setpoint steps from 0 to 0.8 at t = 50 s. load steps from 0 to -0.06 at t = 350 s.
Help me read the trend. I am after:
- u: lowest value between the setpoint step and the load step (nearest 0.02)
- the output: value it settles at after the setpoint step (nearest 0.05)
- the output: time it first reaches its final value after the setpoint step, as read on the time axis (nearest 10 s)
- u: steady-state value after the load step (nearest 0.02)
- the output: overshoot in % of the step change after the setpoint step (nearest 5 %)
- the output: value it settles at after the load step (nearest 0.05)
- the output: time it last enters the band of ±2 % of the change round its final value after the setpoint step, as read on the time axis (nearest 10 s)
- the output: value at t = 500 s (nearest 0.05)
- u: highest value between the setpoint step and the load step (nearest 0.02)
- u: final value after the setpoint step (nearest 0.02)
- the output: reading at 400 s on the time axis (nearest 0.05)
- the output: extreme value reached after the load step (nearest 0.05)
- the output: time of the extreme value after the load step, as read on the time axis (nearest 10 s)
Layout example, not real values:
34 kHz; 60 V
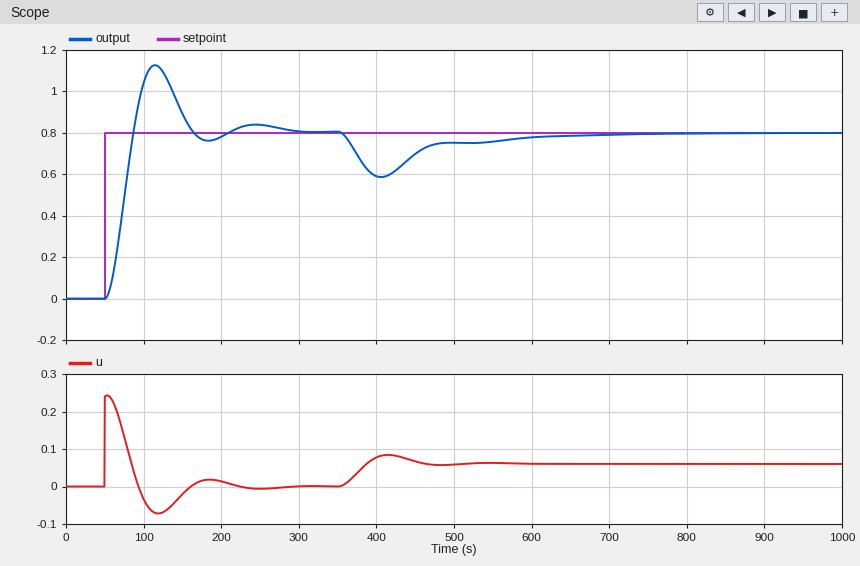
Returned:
-0.08; 0.80; 90 s; 0.06; 40 %; 0.80; 280 s; 0.75; 0.24; 0.00; 0.60; 0.60; 410 s
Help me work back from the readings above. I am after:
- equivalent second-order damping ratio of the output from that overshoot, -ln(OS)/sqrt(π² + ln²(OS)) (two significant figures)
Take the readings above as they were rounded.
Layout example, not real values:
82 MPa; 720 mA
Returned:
0.28
